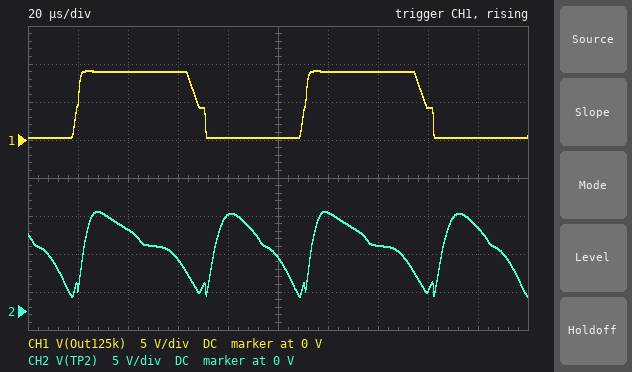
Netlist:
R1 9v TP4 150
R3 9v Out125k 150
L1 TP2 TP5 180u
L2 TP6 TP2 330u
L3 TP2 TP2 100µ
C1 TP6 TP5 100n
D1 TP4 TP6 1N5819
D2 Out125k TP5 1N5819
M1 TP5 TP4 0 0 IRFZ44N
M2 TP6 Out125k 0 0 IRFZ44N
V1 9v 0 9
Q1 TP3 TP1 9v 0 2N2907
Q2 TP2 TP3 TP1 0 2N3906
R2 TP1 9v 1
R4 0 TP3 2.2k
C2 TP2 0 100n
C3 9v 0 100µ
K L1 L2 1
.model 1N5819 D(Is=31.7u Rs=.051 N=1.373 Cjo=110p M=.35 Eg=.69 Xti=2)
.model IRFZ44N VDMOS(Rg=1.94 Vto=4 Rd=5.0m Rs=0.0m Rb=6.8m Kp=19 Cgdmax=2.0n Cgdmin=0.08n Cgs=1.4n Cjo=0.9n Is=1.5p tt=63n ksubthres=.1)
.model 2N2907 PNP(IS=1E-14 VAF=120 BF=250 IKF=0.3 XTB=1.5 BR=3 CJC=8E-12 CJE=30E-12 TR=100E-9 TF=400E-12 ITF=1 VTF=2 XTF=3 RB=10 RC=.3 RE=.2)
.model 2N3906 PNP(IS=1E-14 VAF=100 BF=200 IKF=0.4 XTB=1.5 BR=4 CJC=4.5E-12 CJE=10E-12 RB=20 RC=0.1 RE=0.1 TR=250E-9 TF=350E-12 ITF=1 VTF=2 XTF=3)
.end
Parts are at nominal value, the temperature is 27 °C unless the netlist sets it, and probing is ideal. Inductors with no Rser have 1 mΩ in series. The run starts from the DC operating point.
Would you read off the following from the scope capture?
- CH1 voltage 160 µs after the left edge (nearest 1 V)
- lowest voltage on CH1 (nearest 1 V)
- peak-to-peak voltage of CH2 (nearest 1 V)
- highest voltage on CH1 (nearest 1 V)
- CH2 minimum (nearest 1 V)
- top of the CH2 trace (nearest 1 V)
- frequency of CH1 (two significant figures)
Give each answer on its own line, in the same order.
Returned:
4 V
0 V
11 V
9 V
2 V
13 V
11 kHz
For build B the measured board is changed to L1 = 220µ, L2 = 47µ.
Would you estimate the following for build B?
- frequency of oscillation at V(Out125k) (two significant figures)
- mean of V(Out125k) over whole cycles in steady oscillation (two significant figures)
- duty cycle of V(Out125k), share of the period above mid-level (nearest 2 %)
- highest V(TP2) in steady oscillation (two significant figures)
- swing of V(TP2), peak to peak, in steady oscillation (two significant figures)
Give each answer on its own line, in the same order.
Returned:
17 kHz
3.4 V
36 %
14 V
13 V
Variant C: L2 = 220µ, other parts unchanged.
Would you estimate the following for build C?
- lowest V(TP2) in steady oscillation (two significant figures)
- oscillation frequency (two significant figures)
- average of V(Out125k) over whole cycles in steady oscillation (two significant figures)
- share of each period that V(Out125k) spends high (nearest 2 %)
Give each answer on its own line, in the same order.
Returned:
2.0 V
13 kHz
4.6 V
48 %
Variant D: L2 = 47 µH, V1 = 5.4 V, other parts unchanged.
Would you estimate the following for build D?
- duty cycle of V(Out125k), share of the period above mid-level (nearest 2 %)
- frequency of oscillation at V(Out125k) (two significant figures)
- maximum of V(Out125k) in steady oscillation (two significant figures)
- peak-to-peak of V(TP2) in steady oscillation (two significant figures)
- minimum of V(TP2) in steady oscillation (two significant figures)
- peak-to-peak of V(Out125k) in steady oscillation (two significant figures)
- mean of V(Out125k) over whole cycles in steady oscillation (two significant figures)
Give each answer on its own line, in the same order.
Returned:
42 %
19 kHz
5.4 V
7.6 V
1.4 V
5.2 V
2.4 V
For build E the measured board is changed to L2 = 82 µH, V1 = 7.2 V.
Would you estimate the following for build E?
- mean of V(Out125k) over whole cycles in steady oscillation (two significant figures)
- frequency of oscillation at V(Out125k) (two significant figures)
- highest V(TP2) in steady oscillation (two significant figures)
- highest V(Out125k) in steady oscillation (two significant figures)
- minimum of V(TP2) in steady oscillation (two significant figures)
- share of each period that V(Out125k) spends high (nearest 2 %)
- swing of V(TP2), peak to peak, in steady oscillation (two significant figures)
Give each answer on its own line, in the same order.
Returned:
3.2 V
17 kHz
11 V
7.2 V
1.7 V
44 %
9.4 V
